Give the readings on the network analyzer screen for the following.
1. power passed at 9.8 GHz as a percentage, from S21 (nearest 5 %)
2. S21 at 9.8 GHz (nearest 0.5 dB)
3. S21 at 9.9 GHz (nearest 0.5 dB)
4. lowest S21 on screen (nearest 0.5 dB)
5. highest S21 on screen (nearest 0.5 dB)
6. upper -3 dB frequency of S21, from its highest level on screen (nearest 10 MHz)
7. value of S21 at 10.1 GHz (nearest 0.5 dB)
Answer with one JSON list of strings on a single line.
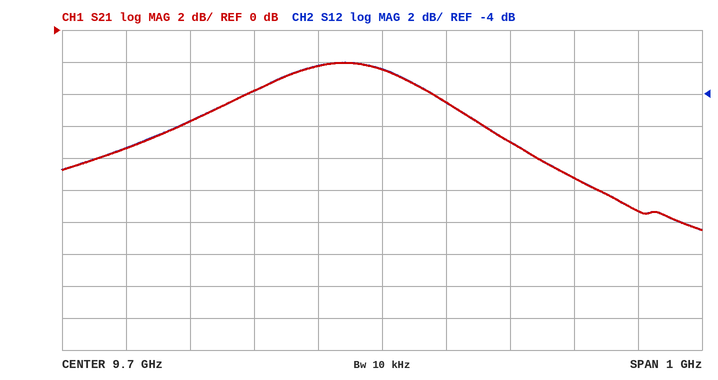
["35 %", "-4.5 dB", "-7.0 dB", "-12.5 dB", "-2.0 dB", "9.82 GHz", "-11.5 dB"]
